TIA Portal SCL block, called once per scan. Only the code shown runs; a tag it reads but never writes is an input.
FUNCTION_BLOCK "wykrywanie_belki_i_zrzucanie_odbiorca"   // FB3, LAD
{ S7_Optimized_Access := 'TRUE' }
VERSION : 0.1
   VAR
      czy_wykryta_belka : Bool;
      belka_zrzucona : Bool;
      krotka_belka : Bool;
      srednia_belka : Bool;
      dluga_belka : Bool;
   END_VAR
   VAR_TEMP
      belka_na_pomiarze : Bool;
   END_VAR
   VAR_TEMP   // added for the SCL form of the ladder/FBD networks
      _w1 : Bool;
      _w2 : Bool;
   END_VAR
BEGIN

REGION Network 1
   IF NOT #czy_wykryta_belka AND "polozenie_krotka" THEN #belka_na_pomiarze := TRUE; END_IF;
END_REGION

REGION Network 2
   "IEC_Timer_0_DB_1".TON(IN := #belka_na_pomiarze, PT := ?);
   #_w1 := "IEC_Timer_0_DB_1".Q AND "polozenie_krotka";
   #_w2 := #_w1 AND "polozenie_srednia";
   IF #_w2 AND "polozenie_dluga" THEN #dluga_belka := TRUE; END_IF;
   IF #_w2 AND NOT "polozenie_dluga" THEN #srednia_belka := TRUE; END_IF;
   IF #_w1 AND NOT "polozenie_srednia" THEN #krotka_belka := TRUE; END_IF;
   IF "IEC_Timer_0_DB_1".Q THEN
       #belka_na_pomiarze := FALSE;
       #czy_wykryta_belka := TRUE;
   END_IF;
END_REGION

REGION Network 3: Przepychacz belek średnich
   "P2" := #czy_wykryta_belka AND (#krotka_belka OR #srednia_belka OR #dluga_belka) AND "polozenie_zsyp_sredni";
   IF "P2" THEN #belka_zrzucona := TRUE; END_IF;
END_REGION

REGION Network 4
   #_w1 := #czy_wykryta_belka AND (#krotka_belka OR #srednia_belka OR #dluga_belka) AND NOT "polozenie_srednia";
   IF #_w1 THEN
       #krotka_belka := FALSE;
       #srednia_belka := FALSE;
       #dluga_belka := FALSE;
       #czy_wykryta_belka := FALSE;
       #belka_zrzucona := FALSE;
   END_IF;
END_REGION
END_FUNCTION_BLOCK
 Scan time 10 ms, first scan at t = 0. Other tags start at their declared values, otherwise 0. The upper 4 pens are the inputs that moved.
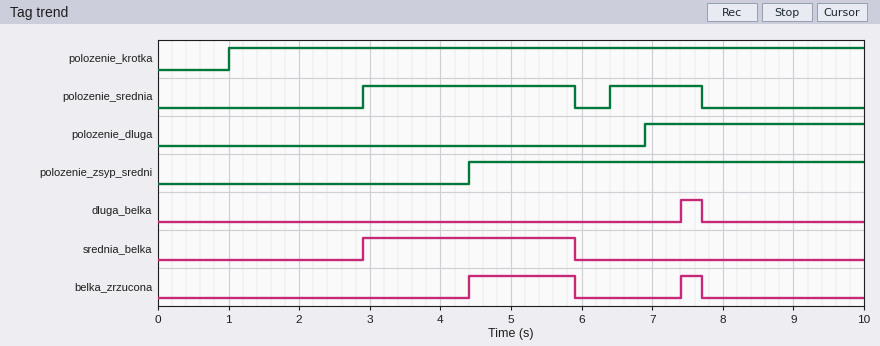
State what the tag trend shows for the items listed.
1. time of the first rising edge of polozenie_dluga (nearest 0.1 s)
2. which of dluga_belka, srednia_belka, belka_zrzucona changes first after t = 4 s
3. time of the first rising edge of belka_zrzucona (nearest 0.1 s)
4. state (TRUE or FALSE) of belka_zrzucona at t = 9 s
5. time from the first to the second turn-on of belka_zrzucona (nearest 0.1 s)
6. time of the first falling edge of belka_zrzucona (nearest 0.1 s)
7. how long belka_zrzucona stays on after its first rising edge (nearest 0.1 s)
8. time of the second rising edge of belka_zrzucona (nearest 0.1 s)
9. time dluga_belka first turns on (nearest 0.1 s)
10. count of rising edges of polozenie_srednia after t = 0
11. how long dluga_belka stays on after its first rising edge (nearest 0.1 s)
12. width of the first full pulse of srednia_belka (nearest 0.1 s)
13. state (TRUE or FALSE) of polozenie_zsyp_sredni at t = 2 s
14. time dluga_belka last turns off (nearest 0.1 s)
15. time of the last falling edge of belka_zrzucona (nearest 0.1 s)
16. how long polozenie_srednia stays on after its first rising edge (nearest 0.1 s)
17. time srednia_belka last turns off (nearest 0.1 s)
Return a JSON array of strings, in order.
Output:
["6.9 s", "belka_zrzucona", "4.4 s", "FALSE", "3.0 s", "5.9 s", "1.5 s", "7.4 s", "7.4 s", "2", "0.3 s", "3.0 s", "FALSE", "7.7 s", "7.7 s", "3.0 s", "5.9 s"]
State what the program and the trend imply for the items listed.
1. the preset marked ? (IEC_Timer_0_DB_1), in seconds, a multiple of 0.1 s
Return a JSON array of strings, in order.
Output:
["1.5 s"]
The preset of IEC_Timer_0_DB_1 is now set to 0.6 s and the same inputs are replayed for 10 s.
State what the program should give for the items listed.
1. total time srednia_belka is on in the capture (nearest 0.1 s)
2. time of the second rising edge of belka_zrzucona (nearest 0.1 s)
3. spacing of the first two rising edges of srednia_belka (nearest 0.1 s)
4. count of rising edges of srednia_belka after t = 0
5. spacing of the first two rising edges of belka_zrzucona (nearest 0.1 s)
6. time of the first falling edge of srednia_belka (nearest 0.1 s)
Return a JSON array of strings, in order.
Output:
["4.2 s", "6.5 s", "3.6 s", "2", "2.1 s", "5.9 s"]
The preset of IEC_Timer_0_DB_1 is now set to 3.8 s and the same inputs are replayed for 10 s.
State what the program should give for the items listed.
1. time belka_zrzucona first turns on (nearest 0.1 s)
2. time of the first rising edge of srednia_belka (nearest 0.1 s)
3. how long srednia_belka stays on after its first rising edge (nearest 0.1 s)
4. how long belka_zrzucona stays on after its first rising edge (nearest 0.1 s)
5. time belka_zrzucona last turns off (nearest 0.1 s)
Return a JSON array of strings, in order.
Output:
["4.8 s", "4.8 s", "1.1 s", "1.1 s", "5.9 s"]
